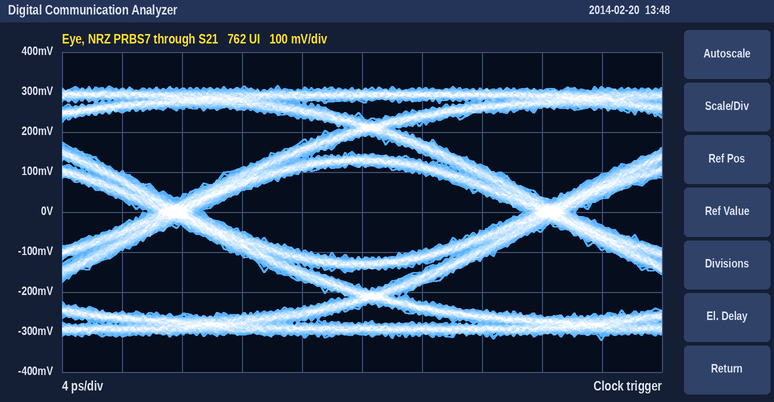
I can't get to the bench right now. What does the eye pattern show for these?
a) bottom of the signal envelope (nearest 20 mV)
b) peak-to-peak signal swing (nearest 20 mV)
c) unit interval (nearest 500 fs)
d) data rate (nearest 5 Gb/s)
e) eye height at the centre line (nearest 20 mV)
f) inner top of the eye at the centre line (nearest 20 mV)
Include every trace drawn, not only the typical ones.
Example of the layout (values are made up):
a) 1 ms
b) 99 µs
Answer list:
a) -320 mV
b) 640 mV
c) 25.0 ps
d) 40 Gb/s
e) 240 mV
f) 120 mV
